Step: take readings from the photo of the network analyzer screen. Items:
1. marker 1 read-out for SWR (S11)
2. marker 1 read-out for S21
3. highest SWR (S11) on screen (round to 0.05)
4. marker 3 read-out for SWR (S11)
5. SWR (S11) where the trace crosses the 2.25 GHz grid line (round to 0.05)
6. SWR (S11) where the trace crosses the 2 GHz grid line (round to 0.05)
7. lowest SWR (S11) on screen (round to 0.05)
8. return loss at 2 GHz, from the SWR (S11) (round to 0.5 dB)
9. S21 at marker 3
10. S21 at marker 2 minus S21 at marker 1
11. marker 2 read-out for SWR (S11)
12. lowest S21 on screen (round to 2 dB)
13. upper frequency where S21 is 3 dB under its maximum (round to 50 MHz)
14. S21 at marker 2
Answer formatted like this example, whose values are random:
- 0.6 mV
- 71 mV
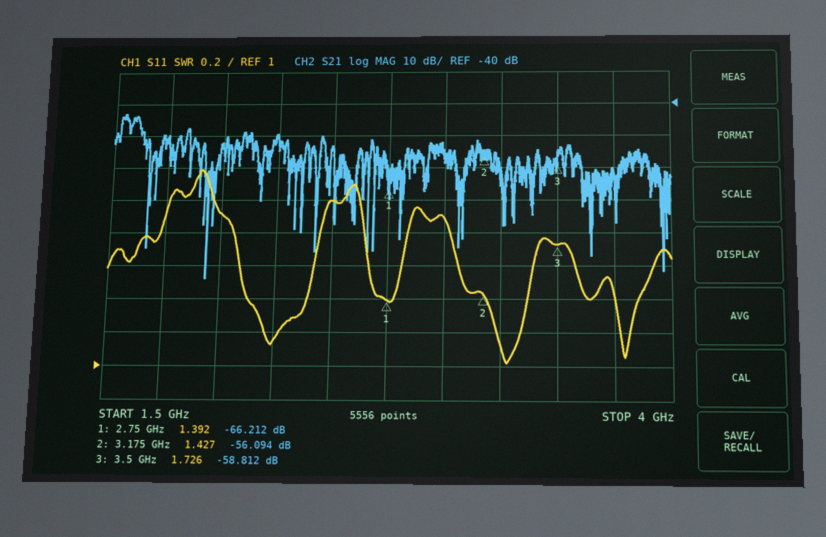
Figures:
- 1.392
- -66.212 dB
- 2.20
- 1.726
- 1.15
- 1.90
- 1.00
- 10.0 dB
- -58.812 dB
- 10.118 dB
- 1.427
- -94 dB
- 1.55 GHz
- -56.094 dB
